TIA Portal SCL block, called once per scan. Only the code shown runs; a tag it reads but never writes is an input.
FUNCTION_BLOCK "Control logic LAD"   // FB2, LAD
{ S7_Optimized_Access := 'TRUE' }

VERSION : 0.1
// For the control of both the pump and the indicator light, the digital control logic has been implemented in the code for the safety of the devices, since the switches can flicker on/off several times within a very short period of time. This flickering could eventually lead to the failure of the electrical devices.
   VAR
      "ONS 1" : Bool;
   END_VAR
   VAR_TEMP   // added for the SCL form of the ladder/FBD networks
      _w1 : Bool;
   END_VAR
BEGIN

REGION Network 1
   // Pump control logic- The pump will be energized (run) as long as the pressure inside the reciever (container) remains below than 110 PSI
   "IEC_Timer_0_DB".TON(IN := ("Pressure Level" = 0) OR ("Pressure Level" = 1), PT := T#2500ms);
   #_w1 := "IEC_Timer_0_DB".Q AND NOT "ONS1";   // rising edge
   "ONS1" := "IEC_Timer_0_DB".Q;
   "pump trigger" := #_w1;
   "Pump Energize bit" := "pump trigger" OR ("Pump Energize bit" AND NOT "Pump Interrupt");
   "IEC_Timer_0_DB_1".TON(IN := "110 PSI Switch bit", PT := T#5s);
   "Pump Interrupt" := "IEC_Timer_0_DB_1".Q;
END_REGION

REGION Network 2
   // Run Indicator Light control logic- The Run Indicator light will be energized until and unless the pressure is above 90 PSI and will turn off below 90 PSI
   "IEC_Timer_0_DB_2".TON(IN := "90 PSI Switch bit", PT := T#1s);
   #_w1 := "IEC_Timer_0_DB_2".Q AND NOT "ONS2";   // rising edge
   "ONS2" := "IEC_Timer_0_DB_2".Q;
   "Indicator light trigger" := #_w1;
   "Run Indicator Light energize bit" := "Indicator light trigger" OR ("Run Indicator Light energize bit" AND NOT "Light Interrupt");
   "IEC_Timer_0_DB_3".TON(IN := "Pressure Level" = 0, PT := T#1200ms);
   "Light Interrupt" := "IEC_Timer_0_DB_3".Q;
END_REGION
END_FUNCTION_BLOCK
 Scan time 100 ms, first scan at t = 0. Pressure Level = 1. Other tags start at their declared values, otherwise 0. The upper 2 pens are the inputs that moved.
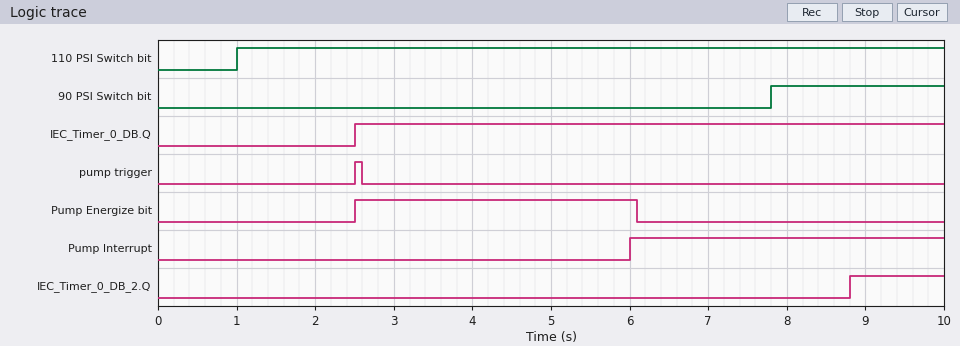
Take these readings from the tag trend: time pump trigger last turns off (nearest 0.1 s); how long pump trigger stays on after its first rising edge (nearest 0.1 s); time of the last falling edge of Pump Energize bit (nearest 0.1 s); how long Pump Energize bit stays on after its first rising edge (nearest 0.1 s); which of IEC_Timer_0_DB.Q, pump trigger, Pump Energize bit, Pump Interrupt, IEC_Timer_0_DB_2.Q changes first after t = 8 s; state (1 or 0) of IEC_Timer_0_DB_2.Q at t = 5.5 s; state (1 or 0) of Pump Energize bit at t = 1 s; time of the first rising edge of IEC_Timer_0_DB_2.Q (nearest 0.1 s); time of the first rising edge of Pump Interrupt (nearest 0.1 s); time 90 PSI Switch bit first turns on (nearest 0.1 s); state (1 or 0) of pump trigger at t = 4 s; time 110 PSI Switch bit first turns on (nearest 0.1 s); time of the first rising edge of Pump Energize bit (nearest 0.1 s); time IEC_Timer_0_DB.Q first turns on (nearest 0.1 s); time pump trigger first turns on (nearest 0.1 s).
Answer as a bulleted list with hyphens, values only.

- 2.6 s
- 0.1 s
- 6.1 s
- 3.6 s
- IEC_Timer_0_DB_2.Q
- 0
- 0
- 8.8 s
- 6.0 s
- 7.8 s
- 0
- 1.0 s
- 2.5 s
- 2.5 s
- 2.5 s
